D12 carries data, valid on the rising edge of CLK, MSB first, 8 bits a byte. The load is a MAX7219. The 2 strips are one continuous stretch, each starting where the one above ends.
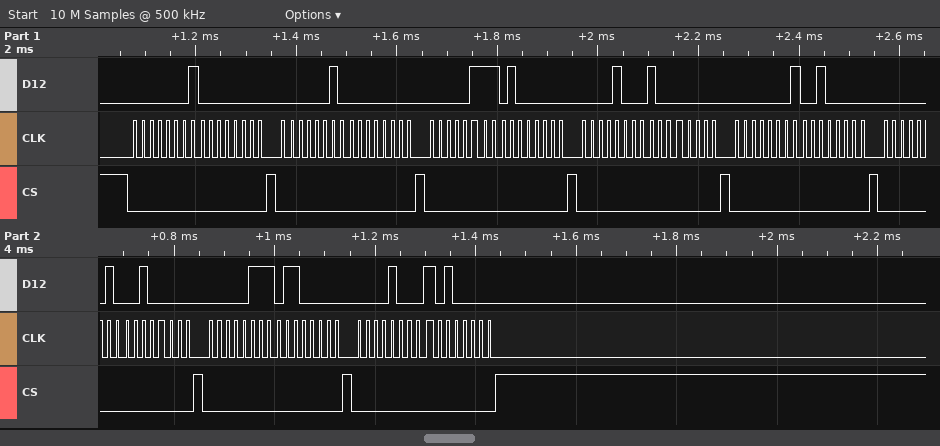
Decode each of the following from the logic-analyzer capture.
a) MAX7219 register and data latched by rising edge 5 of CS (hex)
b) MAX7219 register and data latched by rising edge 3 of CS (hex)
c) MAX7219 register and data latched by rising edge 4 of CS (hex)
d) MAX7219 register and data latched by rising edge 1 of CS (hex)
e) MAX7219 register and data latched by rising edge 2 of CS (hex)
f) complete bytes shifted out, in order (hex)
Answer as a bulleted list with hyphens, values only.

- register 0x1, data 0x20
- register 0x7, data 0x40
- register 0x8, data 0x80
- register 0x1, data 0x00
- register 0x2, data 0x00
- 01 00 02 00 07 40 08 80 01 20 02 20 07 60 08 A0
